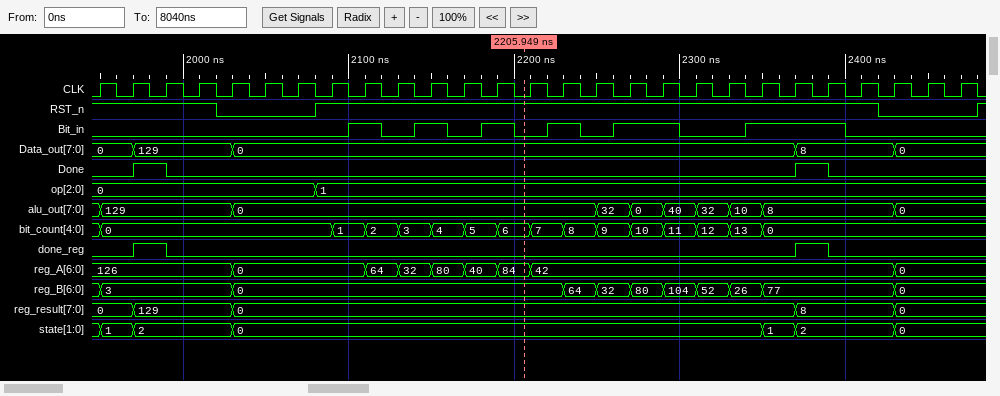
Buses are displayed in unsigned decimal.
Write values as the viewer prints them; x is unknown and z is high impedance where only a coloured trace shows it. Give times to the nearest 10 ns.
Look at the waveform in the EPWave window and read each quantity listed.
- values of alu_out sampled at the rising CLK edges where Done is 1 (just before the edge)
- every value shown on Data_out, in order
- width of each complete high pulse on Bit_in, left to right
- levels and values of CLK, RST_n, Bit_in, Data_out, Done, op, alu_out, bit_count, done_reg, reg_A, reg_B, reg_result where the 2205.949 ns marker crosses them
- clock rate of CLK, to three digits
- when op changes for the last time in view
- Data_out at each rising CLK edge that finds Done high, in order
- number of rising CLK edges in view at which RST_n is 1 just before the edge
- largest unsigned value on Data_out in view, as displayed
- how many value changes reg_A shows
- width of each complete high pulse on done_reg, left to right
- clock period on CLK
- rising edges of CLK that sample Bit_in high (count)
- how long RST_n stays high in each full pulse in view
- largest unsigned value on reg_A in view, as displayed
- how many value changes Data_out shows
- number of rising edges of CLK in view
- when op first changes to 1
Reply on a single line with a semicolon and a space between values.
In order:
129, 8; 0, 129, 0, 8, 0; 20 ns, 20 ns, 20 ns, 20 ns, 40 ns, 60 ns; CLK=0, RST_n=1, Bit_in=0, Data_out=0, Done=0, op=1, alu_out=0, bit_count=6, done_reg=0, reg_A=84, reg_B=0, reg_result=0; 50.0 MHz; 2080 ns; 129, 8; 21; 129; 8; 20 ns, 20 ns; 20 ns; 9; 340 ns; 126; 4; 27; 2080 ns
